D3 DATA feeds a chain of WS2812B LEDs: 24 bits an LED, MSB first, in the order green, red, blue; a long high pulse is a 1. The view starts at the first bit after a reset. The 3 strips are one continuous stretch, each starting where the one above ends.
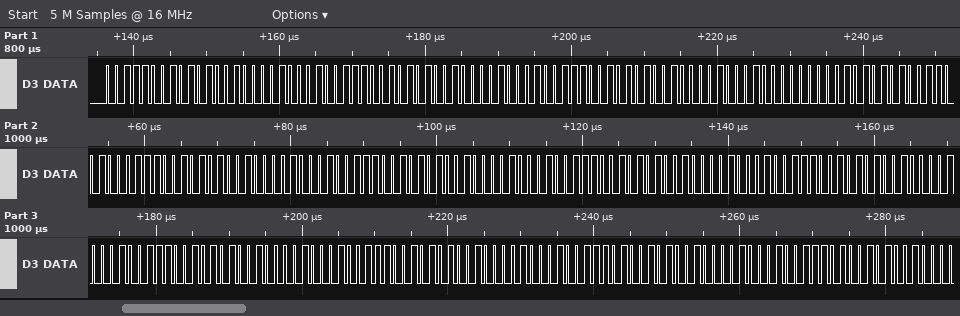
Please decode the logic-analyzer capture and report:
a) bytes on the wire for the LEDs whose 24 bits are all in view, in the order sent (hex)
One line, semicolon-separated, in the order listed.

39 52 11 39 52 11 39 52 11 00 55 32 39 52 11 39 52 11 39 52 11 39 52 11 39 52 11 39 52 11 3A 52 11
